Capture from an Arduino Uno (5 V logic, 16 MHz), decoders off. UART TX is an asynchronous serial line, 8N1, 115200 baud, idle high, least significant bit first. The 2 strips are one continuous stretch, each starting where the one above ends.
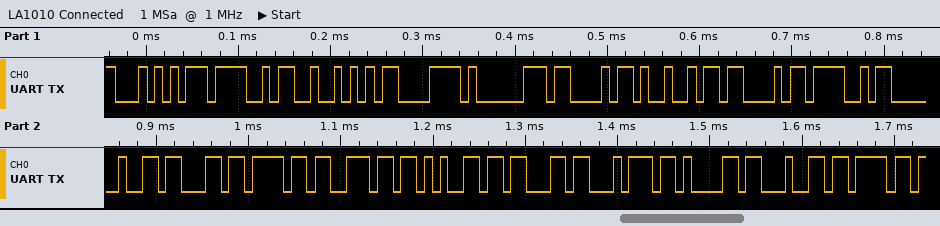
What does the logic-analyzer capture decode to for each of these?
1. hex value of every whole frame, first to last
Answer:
0x54 0x4F 0x52 0xC3 0x81 0x43 0x49 0x43 0x4F 0x20 0x63 0x6F 0x6E 0x65 0x63 0x74 0x61 0x64 0x6F
